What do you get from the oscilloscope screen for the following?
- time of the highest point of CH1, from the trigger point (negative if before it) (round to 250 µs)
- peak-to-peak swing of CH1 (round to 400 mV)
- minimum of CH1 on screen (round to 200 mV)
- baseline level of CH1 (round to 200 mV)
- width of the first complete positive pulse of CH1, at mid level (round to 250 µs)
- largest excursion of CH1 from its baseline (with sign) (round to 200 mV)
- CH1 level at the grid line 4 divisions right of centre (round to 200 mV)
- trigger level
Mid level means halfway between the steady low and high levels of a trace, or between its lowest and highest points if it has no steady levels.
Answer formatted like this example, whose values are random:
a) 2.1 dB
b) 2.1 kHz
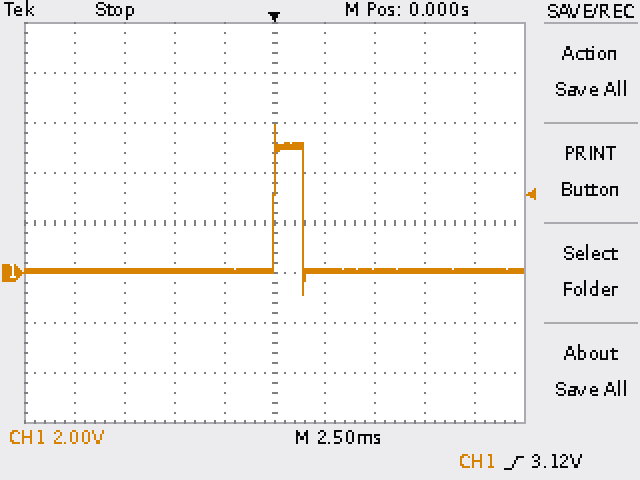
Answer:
a) 0.00 ms
b) 6.8 V
c) -800 mV
d) 0.0 V
e) 1.50 ms
f) +5.8 V
g) 0.0 V
h) 3.12 V
